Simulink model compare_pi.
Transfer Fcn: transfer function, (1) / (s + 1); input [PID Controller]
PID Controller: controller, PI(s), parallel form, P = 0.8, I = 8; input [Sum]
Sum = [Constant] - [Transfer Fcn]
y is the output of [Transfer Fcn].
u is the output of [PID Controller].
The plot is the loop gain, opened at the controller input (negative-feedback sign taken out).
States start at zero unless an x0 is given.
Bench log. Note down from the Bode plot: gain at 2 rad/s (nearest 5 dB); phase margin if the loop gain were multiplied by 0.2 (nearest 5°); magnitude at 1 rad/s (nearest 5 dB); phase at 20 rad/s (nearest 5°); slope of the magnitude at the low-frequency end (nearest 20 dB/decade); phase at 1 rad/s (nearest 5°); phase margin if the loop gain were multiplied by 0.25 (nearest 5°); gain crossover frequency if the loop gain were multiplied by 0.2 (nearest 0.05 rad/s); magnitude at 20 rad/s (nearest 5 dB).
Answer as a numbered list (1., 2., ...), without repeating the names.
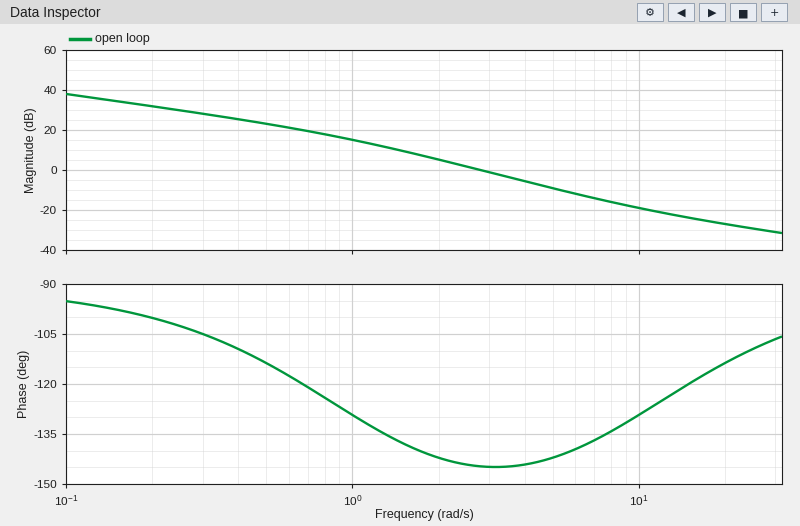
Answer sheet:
1. 5 dB
2. 50°
3. 15 dB
4. -115°
5. -20 dB/decade
6. -130°
7. 45°
8. 1.10 rad/s
9. -25 dB
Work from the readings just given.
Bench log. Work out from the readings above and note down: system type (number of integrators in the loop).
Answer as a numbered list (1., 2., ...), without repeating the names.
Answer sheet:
1. 1
